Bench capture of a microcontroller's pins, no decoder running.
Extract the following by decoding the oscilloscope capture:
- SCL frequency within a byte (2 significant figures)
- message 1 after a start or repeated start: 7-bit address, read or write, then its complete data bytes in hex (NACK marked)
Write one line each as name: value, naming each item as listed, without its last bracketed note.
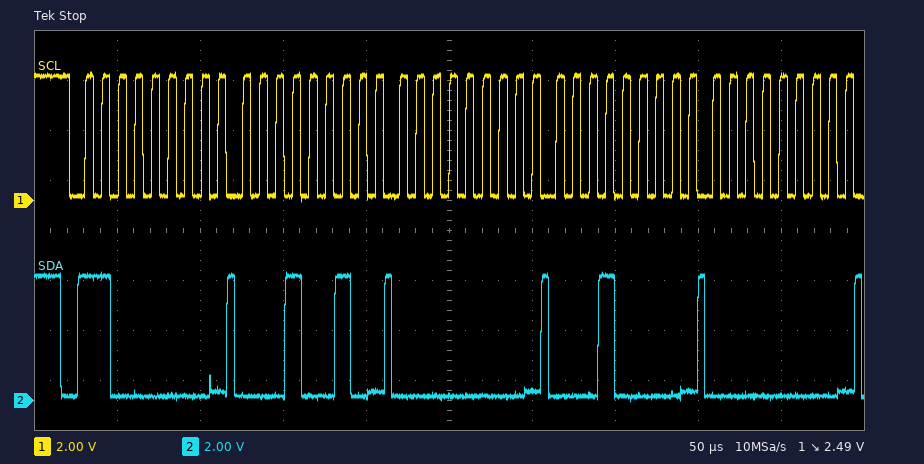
SCL frequency within a byte: 100 kHz
message 1 after a start or repeated start: 7-bit address, read or write, then its complete data bytes in hex: 0x60 write: 12 00 10 00
